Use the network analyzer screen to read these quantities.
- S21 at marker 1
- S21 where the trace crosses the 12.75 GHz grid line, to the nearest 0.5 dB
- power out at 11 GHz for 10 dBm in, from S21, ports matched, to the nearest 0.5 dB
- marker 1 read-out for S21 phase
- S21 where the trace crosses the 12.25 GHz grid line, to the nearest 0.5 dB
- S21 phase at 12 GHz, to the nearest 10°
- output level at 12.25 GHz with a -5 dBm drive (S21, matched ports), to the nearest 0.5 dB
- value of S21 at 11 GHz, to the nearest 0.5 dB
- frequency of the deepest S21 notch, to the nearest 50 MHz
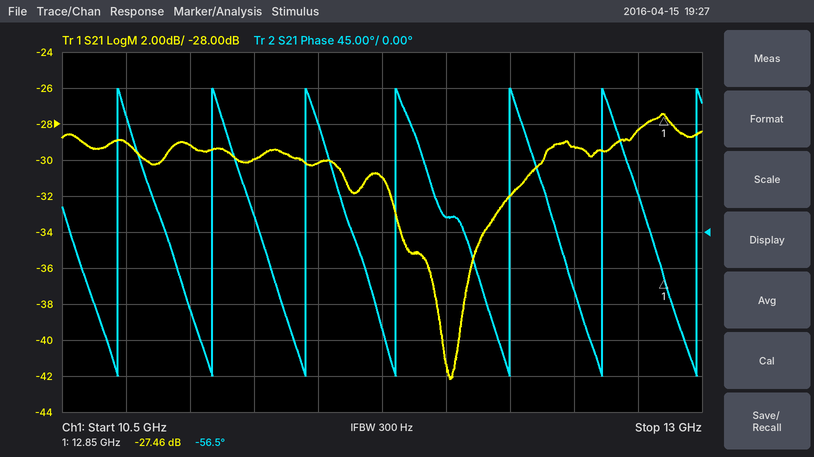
-27.46 dB
-28.5 dB
-19.0 dBm
-56.5°
-32.0 dB
20°
-37.0 dBm
-29.0 dB
12.00 GHz
